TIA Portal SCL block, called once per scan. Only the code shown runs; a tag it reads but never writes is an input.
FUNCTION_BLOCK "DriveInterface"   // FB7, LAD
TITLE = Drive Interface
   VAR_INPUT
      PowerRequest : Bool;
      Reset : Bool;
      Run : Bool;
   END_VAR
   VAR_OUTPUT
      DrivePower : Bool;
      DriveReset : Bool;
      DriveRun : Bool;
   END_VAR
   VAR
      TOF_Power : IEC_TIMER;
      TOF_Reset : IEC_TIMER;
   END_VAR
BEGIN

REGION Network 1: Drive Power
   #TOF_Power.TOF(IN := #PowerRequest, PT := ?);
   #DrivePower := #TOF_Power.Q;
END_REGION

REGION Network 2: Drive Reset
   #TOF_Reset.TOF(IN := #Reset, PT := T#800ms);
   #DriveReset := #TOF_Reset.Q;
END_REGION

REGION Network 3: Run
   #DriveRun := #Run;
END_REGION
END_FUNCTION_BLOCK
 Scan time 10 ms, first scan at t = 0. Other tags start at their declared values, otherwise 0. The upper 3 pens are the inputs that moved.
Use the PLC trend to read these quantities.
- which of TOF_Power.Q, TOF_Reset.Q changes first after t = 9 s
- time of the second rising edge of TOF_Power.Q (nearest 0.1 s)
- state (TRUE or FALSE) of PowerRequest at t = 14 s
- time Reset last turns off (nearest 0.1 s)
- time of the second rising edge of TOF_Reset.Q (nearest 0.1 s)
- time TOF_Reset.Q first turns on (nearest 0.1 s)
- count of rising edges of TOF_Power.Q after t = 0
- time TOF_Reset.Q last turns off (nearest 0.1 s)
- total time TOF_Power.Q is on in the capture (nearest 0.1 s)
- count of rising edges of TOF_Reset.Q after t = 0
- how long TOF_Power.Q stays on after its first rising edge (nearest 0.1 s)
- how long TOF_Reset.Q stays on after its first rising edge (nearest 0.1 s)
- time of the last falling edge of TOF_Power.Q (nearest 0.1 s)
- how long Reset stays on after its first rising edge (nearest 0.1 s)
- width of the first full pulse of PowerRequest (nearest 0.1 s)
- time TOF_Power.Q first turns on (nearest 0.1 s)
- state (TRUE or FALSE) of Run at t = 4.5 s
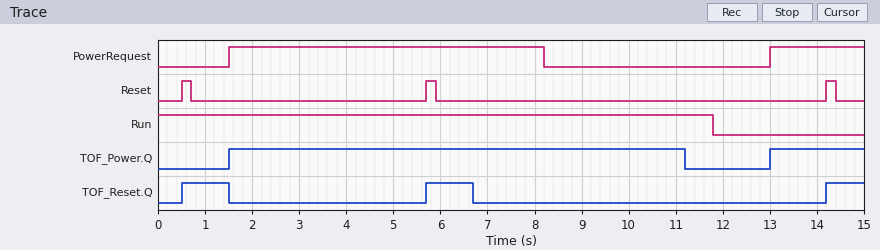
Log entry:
TOF_Power.Q
13.0 s
TRUE
14.4 s
5.7 s
0.5 s
2
6.7 s
11.7 s
3
9.7 s
1.0 s
11.2 s
0.2 s
6.7 s
1.5 s
TRUE
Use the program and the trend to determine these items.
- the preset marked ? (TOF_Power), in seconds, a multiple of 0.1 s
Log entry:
3.0 s
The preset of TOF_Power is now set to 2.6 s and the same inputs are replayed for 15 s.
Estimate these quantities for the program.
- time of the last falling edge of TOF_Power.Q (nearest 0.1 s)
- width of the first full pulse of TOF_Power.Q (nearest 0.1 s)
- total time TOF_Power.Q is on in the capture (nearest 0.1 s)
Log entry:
10.8 s
9.3 s
11.3 s
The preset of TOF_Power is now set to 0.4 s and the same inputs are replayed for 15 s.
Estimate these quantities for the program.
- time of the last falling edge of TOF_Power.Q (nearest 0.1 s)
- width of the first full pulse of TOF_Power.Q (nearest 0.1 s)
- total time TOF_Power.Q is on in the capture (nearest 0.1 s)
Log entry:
8.6 s
7.1 s
9.1 s
